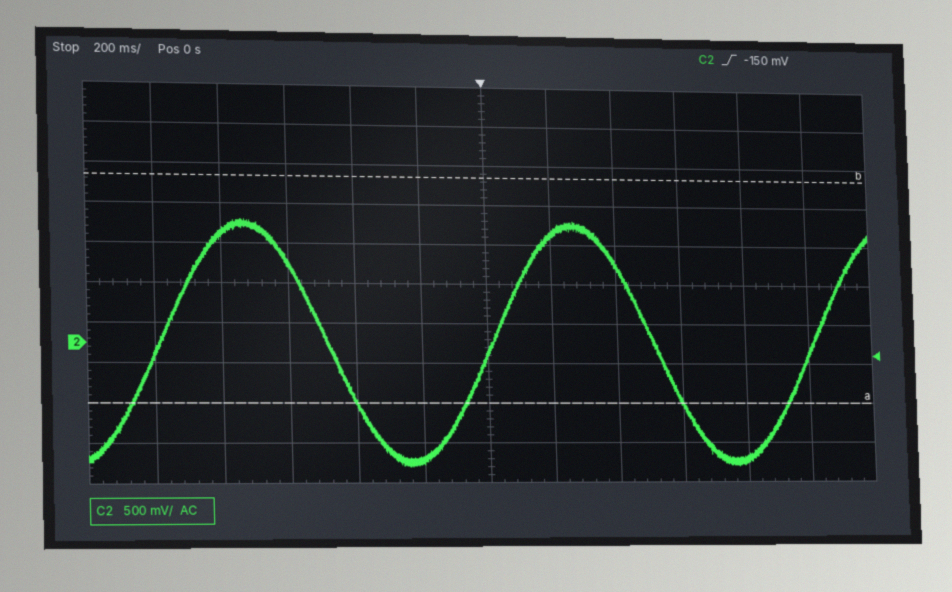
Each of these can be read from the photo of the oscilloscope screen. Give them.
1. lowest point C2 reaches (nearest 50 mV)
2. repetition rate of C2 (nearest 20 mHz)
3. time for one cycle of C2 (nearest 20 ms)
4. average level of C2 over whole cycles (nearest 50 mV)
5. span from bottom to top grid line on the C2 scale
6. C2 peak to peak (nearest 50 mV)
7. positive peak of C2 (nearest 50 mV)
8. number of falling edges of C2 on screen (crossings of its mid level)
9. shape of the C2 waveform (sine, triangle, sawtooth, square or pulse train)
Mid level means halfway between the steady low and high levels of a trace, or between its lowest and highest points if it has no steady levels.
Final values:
-1.55 V
1.00 Hz
1.00 s
0 mV
5 V
3.10 V
1.55 V
2
sine
